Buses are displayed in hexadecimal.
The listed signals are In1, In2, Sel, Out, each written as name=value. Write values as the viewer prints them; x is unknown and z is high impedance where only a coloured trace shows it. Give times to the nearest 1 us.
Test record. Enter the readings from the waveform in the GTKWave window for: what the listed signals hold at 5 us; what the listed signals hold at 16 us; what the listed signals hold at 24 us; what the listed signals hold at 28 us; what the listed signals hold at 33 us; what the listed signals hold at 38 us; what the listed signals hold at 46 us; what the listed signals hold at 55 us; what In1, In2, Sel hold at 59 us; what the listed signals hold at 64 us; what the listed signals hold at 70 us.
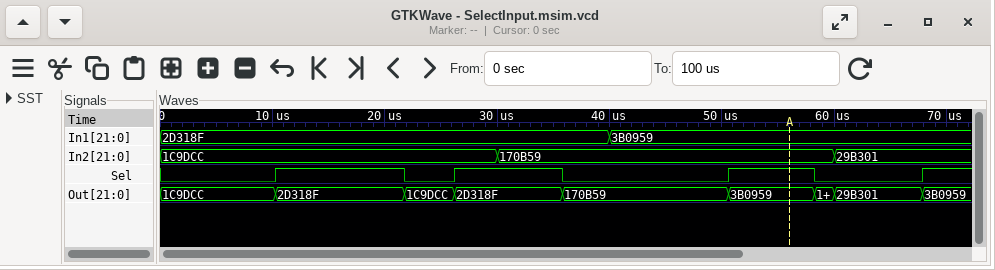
In1=2D318F, In2=1C9DCC, Sel=0, Out=1C9DCC
In1=2D318F, In2=1C9DCC, Sel=1, Out=2D318F
In1=2D318F, In2=1C9DCC, Sel=0, Out=1C9DCC
In1=2D318F, In2=1C9DCC, Sel=1, Out=2D318F
In1=2D318F, In2=170B59, Sel=1, Out=2D318F
In1=2D318F, In2=170B59, Sel=0, Out=170B59
In1=3B0959, In2=170B59, Sel=0, Out=170B59
In1=3B0959, In2=170B59, Sel=1, Out=3B0959
In1=3B0959, In2=170B59, Sel=0
In1=3B0959, In2=29B301, Sel=0, Out=29B301
In1=3B0959, In2=29B301, Sel=1, Out=3B0959
